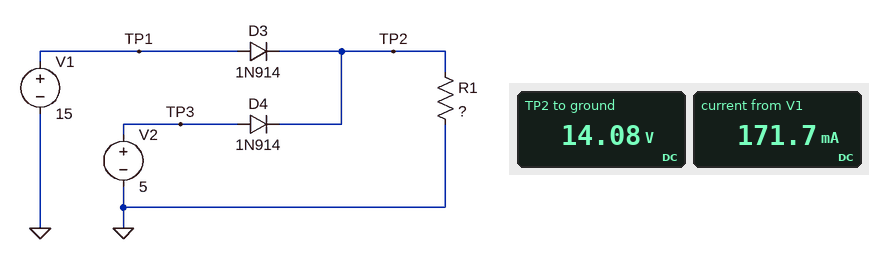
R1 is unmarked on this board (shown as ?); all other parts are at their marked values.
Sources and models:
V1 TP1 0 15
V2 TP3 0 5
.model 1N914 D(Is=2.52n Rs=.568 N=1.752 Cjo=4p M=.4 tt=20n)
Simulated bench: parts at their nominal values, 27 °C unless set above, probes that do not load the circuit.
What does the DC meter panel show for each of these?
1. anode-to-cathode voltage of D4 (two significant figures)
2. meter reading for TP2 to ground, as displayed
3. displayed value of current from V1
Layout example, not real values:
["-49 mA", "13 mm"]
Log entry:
["-9.1 V", "14.08 V", "171.7 mA"]
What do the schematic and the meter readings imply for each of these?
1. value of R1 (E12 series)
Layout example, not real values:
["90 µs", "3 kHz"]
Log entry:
["82 Ω"]
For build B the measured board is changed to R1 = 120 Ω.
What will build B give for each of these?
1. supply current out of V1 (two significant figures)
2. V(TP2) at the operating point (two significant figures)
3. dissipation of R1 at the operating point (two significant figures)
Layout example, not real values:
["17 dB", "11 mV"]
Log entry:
["120 mA", "14 V", "1.7 W"]
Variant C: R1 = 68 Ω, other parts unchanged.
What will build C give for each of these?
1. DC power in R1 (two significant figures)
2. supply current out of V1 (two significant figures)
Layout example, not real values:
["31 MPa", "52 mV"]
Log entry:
["2.9 W", "210 mA"]
